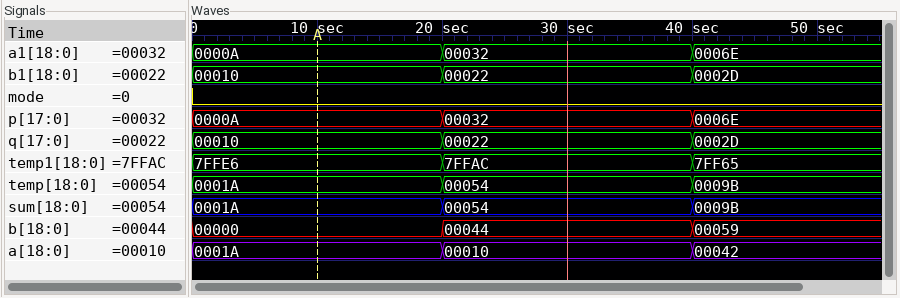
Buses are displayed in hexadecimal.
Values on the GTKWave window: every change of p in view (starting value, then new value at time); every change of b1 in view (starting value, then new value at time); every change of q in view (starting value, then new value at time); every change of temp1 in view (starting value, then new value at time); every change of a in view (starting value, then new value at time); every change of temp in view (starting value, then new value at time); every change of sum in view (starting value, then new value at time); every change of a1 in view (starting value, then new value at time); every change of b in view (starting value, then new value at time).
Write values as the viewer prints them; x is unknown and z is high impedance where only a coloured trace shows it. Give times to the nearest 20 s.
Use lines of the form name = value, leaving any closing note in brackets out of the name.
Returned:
every change of p in view = 0000A, 00032 at 20 s, 0006E at 40 s
every change of b1 in view = 00010, 00022 at 20 s, 0002D at 40 s
every change of q in view = 00010, 00022 at 20 s, 0002D at 40 s
every change of temp1 in view = 7FFE6, 7FFAC at 20 s, 7FF65 at 40 s
every change of a in view = 0001A, 00010 at 20 s, 00042 at 40 s
every change of temp in view = 0001A, 00054 at 20 s, 0009B at 40 s
every change of sum in view = 0001A, 00054 at 20 s, 0009B at 40 s
every change of a1 in view = 0000A, 00032 at 20 s, 0006E at 40 s
every change of b in view = 00000, 00044 at 20 s, 00059 at 40 s
